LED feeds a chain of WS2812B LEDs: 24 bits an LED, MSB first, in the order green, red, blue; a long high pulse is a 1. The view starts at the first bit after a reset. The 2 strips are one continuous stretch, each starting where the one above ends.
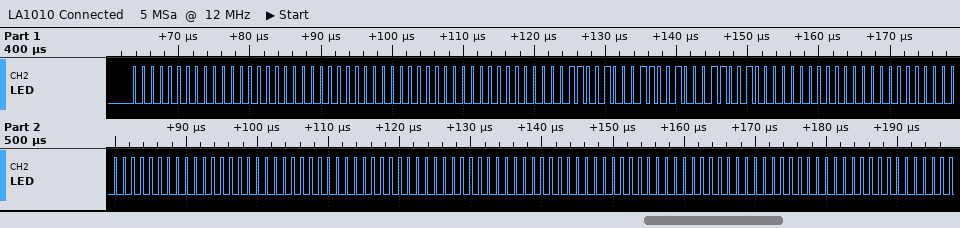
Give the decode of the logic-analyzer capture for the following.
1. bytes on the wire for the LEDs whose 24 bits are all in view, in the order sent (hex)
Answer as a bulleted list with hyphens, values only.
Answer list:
- 00 00 00 00 00 00 64 64 64 00 00 00 00 00 00 00 00 00 00 00 00
